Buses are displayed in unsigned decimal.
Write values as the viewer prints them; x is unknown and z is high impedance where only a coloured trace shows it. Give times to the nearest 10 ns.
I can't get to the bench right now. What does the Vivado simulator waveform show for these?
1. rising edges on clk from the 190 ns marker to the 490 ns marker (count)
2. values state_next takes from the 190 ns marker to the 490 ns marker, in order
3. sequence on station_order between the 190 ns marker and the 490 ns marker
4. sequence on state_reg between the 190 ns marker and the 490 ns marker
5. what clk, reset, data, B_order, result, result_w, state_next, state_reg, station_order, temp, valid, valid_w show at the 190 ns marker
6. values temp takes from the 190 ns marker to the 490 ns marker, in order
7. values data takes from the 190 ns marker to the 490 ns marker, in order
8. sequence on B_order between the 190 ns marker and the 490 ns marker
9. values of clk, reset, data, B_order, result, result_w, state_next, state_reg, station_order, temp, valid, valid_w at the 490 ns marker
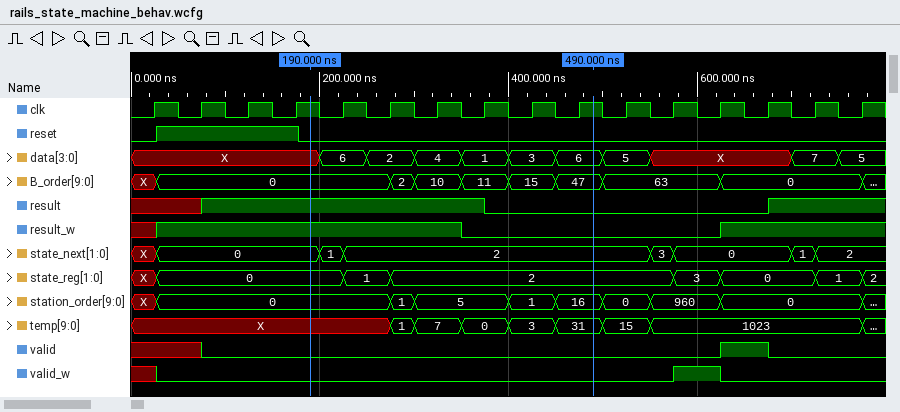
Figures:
6
0, 1, 2
0, 1, 5, 1, 16
0, 1, 2
clk=1, reset=0, data=X, B_order=0, result=1, result_w=1, state_next=0, state_reg=0, station_order=0, temp=X, valid=0, valid_w=0
X, 1, 7, 0, 3, 31
X, 6, 2, 4, 1, 3, 6
0, 2, 10, 11, 15, 47
clk=1, reset=0, data=6, B_order=47, result=0, result_w=0, state_next=2, state_reg=2, station_order=16, temp=31, valid=0, valid_w=0
